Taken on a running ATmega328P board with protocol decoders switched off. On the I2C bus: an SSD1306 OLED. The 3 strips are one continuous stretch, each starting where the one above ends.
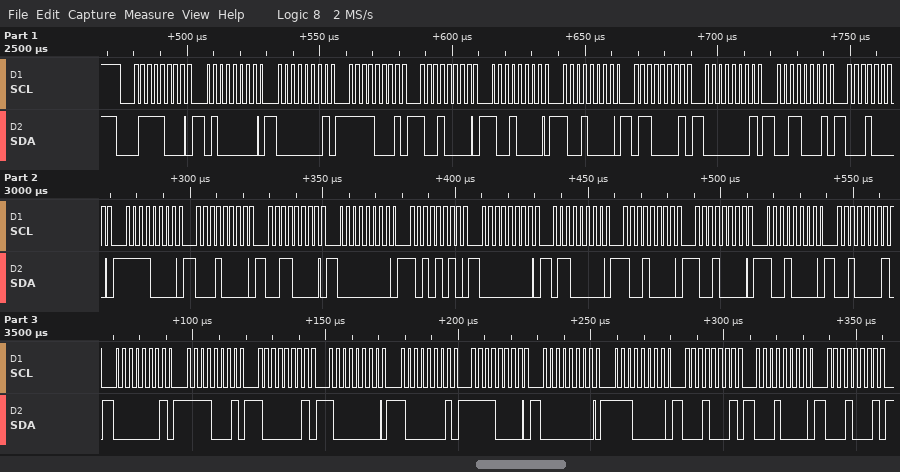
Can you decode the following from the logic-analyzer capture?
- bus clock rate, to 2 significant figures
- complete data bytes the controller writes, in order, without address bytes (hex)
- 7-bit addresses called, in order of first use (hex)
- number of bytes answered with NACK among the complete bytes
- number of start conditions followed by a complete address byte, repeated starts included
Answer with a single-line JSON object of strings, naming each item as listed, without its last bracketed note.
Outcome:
{"bus clock rate, to 2 significant figures": "400 kHz", "complete data bytes the controller writes, in order, without address bytes": "40 01 F1 90 90 90 61 01 31 10 F0 10 30 00 AA 00 60 90 90 90 21 01 F1 81 80 81 F0 00 E0 11 10 11", "7-bit addresses called, in order of first use": "0x3C", "number of bytes answered with NACK among the complete bytes": "0", "number of start conditions followed by a complete address byte, repeated starts included": "1"}
